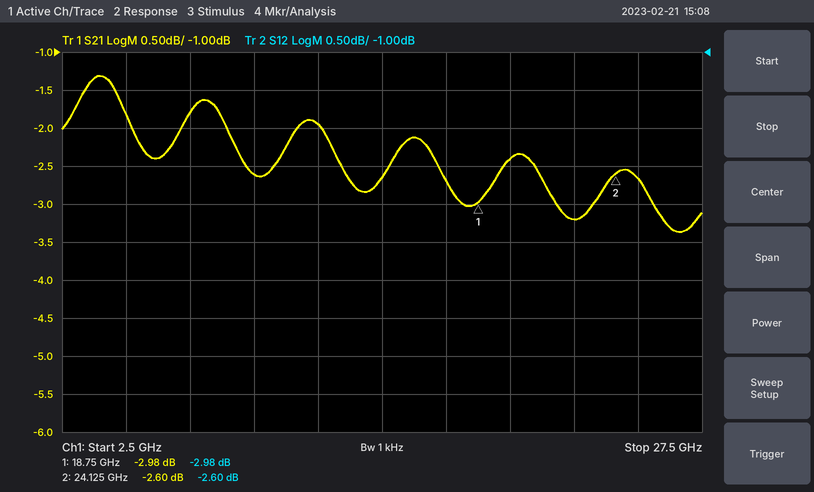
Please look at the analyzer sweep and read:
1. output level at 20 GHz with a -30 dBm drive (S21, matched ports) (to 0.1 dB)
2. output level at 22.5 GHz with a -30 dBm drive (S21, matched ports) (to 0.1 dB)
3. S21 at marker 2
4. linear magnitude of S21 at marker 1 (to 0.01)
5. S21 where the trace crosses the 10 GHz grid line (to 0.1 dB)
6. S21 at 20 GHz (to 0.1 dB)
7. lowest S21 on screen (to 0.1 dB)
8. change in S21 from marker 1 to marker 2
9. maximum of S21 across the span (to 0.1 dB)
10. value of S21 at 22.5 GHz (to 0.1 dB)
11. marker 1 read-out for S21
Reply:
-32.4 dBm
-33.2 dBm
-2.60 dB
0.71
-2.6 dB
-2.4 dB
-3.4 dB
0.38 dB
-1.3 dB
-3.2 dB
-2.98 dB
